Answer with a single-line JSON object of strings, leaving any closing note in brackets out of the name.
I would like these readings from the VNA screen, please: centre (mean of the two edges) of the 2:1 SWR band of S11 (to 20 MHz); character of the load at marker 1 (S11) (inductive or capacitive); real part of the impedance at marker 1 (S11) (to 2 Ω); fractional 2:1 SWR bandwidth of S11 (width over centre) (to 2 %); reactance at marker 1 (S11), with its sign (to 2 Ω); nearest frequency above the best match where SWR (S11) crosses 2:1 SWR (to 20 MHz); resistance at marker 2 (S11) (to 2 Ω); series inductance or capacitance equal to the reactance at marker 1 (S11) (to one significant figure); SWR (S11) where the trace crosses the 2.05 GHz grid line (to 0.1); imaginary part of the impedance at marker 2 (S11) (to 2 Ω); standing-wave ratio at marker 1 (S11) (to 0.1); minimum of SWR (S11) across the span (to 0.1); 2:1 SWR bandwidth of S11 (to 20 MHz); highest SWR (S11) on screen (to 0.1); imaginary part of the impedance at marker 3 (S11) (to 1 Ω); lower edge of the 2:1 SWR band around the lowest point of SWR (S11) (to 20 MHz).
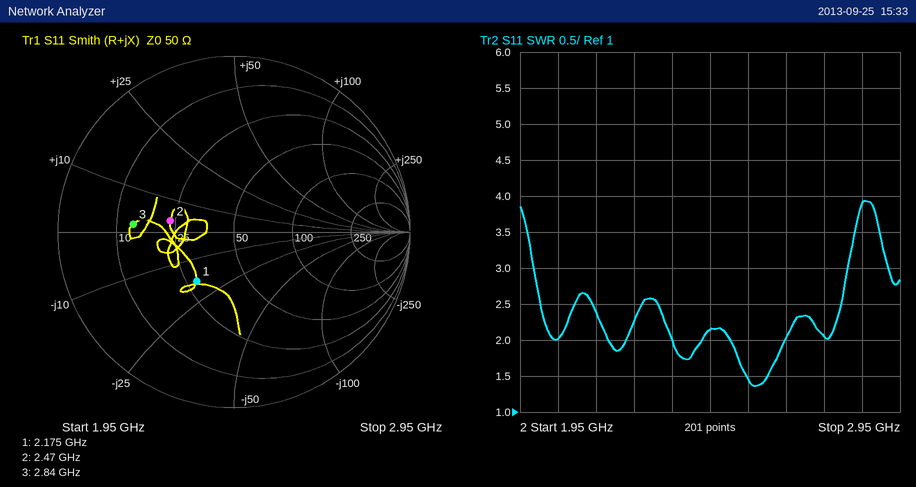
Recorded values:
{"centre (mean of the two edges) of the 2:1 SWR band of S11": "2.58 GHz", "character of the load at marker 1 (S11)": "capacitive", "real part of the impedance at marker 1 (S11)": "28 Ω", "fractional 2:1 SWR bandwidth of S11 (width over centre)": "6 %", "reactance at marker 1 (S11), with its sign": "-18 Ω", "nearest frequency above the best match where SWR (S11) crosses 2:1 SWR": "2.64 GHz", "resistance at marker 2 (S11)": "24 Ω", "series inductance or capacitance equal to the reactance at marker 1 (S11)": "4 pF", "SWR (S11) where the trace crosses the 2.05 GHz grid line": "2.0", "imaginary part of the impedance at marker 2 (S11)": "+4 Ω", "standing-wave ratio at marker 1 (S11)": "2.1", "minimum of SWR (S11) across the span": "1.4", "2:1 SWR bandwidth of S11": "140 MHz", "highest SWR (S11) on screen": "3.9", "imaginary part of the impedance at marker 3 (S11)": "+2 Ω", "lower edge of the 2:1 SWR band around the lowest point of SWR (S11)": "2.50 GHz"}
